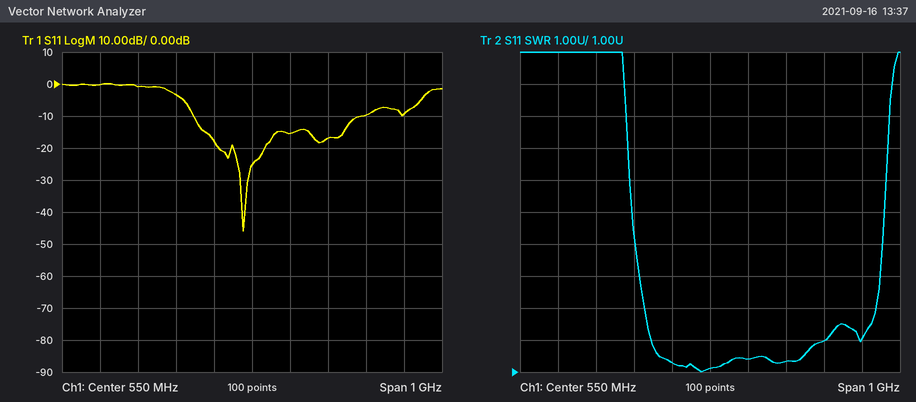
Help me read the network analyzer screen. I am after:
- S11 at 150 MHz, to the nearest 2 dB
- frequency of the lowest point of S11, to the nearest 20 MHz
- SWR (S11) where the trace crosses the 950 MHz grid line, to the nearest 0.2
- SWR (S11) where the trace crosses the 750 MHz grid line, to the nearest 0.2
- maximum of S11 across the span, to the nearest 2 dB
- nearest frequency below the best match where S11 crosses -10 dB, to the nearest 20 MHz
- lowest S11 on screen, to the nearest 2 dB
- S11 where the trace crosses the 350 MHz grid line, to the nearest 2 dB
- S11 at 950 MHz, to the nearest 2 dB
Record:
0 dB
520 MHz
2.0
1.4
0 dB
400 MHz
-46 dB
-4 dB
-10 dB
